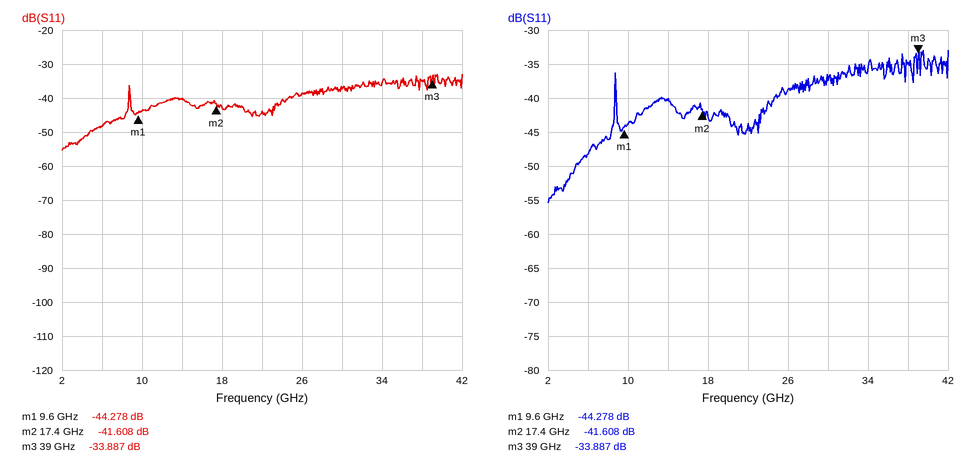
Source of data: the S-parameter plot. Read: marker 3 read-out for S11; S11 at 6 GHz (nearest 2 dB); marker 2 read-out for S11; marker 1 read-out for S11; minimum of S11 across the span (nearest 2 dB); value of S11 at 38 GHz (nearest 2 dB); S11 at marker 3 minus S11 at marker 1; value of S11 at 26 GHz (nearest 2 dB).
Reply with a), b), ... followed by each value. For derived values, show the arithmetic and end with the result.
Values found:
a) -33.887 dB
b) -48 dB
c) -41.608 dB
d) -44.278 dB
e) -56 dB
f) -34 dB
g) -33.887 − (-44.278) = 10.391 dB
h) -38 dB
